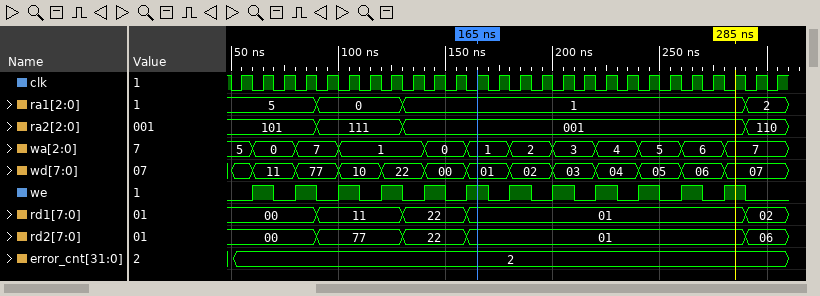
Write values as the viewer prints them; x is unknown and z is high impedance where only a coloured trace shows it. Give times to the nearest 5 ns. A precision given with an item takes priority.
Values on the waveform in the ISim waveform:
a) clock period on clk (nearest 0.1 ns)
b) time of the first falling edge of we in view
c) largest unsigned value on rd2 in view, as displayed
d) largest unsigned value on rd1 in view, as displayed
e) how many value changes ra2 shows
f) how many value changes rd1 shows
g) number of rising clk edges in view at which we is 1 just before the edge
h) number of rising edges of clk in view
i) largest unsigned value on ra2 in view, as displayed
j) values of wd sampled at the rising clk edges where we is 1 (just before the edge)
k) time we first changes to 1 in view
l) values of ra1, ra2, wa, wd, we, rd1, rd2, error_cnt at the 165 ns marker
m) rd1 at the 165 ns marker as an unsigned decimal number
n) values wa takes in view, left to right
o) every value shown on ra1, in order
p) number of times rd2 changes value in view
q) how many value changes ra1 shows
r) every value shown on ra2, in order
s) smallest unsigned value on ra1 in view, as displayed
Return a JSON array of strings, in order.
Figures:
["10 ns", "70 ns", "77", "22", "3", "4", "12", "26", "111", "11, 77, 10, 22, 00, 01, 02, 03, 04, 05, 06, 07", "60 ns", "ra1=1, ra2=001, wa=1, wd=01, we=1, rd1=01, rd2=01, error_cnt=2", "1", "5, 0, 7, 1, 0, 1, 2, 3, 4, 5, 6, 7", "5, 0, 1, 2", "4", "3", "101, 111, 001, 110", "0"]
